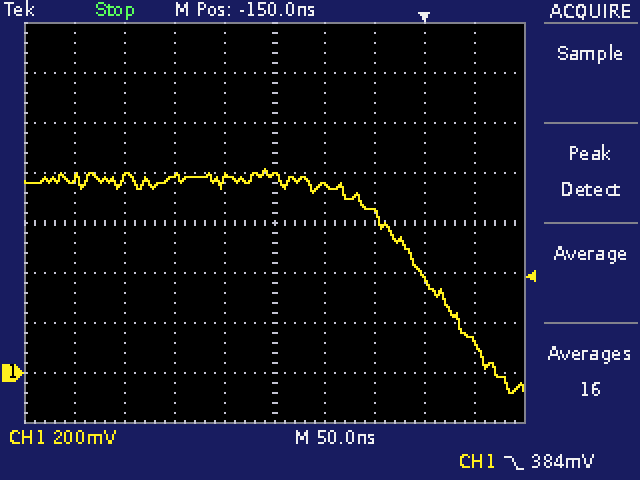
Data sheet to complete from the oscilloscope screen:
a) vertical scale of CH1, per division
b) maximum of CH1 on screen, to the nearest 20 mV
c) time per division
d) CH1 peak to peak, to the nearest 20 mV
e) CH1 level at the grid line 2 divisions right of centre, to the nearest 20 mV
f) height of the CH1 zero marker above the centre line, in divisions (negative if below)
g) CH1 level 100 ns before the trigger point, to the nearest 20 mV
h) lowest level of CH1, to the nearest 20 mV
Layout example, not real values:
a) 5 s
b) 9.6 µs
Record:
a) 200 mV
b) 820 mV
c) 50 ns
d) 900 mV
e) 640 mV
f) -3.0 div
g) 760 mV
h) -80 mV
